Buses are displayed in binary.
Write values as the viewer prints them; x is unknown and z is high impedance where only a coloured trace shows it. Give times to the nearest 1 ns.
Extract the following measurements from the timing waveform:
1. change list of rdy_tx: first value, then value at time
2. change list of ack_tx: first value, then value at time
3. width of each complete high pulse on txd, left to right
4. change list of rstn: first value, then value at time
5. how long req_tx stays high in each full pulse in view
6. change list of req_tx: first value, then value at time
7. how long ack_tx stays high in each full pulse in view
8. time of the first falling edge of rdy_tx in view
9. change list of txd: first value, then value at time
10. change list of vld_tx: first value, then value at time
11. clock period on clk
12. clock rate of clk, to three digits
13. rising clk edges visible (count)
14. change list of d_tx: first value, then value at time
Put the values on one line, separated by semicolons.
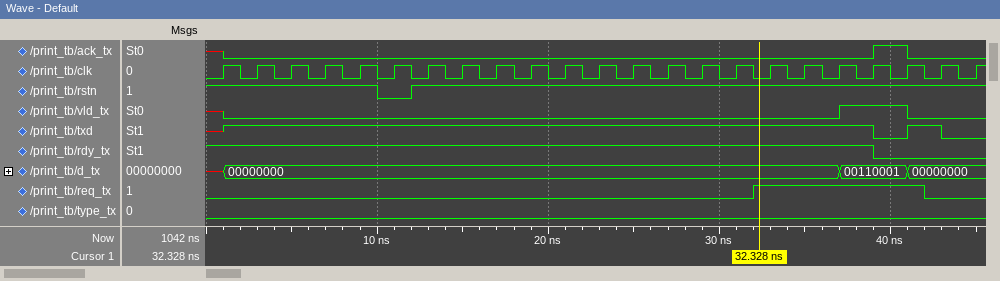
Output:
1, 0 at 39 ns; x, 0 at 1 ns, 1 at 39 ns, 0 at 41 ns; 2 ns; 1, 0 at 10 ns, 1 at 12 ns; 10 ns; 0, 1 at 32 ns, 0 at 42 ns; 2 ns; 39 ns; x, 1 at 1 ns, 0 at 39 ns, 1 at 41 ns, 0 at 43 ns; x, 0 at 1 ns, 1 at 37 ns, 0 at 41 ns; 2 ns; 500 MHz; 23; x, 00000000 at 1 ns, 00110001 at 37 ns, 00000000 at 41 ns
